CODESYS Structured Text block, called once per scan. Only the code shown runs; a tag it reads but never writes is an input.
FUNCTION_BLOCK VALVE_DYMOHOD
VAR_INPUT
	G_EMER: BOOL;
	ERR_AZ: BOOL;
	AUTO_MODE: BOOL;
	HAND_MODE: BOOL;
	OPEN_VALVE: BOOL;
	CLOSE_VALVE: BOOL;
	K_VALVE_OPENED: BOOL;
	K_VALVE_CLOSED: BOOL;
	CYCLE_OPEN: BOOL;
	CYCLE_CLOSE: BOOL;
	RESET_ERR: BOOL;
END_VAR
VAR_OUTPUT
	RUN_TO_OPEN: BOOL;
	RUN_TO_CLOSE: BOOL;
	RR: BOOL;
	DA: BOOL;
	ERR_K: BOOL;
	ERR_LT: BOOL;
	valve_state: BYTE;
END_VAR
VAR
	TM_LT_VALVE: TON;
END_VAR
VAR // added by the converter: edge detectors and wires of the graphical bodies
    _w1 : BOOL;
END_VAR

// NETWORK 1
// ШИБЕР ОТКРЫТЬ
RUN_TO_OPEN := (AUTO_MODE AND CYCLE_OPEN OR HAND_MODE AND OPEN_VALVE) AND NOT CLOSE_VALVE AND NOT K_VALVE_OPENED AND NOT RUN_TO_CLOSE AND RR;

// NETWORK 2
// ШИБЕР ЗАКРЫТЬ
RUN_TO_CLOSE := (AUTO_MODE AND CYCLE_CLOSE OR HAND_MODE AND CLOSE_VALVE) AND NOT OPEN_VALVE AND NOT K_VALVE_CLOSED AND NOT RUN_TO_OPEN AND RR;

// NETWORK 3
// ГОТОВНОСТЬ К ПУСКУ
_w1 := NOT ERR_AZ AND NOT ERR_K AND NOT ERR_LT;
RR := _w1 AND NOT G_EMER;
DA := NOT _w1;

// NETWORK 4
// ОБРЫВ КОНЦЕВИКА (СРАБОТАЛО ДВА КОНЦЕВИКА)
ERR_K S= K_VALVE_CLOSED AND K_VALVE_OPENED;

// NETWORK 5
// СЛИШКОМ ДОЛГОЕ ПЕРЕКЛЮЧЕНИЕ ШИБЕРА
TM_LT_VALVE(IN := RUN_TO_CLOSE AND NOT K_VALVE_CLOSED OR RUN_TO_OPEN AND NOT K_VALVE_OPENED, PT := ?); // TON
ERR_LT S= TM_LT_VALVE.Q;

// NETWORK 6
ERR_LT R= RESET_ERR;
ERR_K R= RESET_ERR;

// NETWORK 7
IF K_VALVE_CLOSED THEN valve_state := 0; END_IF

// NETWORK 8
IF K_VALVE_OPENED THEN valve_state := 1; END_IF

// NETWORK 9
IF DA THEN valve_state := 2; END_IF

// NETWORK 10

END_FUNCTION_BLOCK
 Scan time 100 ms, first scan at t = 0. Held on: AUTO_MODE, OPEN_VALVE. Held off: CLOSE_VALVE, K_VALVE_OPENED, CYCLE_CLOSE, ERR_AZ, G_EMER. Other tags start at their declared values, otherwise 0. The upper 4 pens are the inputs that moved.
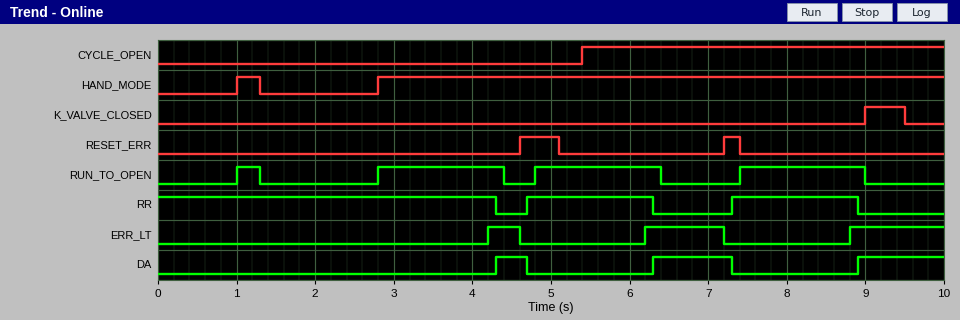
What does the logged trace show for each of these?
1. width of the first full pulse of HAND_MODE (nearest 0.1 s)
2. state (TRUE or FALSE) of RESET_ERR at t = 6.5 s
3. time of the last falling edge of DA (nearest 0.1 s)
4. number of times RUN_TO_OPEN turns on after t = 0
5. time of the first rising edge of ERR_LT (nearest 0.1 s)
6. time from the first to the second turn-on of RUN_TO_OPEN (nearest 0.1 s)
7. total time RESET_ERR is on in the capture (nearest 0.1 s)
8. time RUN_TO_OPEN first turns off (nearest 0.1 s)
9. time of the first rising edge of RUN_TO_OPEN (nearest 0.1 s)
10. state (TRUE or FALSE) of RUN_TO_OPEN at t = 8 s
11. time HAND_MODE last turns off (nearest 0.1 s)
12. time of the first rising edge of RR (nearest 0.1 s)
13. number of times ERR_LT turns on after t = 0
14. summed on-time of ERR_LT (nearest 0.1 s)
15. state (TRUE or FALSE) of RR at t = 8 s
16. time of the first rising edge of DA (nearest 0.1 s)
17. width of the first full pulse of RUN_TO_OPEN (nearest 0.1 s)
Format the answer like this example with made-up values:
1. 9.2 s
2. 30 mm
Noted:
1. 0.3 s
2. FALSE
3. 7.3 s
4. 4
5. 4.2 s
6. 1.8 s
7. 0.7 s
8. 1.3 s
9. 1.0 s
10. TRUE
11. 1.3 s
12. 4.7 s
13. 3
14. 2.6 s
15. TRUE
16. 4.3 s
17. 0.3 s
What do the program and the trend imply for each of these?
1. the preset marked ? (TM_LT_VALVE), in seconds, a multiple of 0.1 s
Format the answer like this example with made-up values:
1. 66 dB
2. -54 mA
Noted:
1. 1.4 s
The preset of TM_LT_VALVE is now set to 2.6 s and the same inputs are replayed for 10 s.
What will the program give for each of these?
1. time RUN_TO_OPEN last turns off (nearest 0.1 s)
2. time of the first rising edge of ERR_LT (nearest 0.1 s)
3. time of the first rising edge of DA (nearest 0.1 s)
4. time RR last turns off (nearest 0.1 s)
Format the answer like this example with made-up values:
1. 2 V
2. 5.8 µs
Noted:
1. 5.6 s
2. 5.4 s
3. 5.5 s
4. 5.5 s
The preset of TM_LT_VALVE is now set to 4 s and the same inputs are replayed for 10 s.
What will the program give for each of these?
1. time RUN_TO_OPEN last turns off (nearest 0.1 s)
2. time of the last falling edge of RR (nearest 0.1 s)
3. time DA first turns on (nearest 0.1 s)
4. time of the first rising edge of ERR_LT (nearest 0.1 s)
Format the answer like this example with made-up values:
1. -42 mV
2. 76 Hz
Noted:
1. 7.0 s
2. 6.9 s
3. 6.9 s
4. 6.8 s
